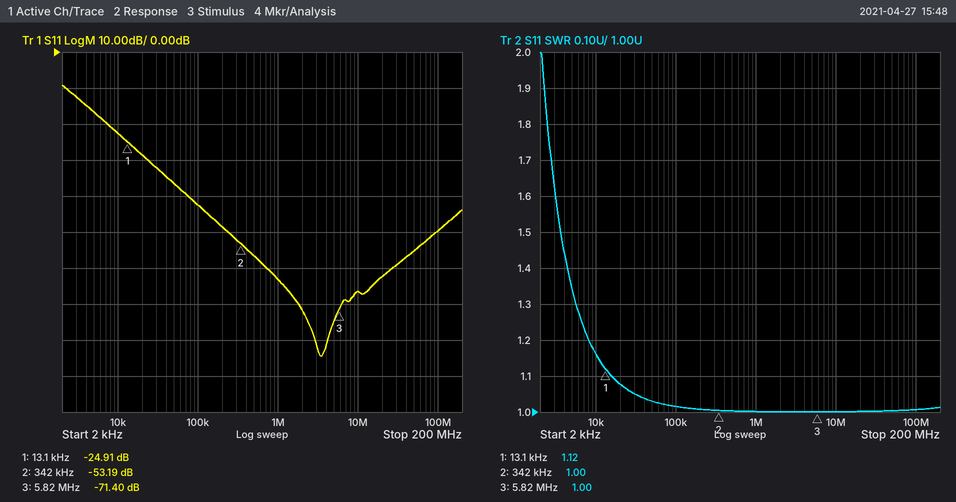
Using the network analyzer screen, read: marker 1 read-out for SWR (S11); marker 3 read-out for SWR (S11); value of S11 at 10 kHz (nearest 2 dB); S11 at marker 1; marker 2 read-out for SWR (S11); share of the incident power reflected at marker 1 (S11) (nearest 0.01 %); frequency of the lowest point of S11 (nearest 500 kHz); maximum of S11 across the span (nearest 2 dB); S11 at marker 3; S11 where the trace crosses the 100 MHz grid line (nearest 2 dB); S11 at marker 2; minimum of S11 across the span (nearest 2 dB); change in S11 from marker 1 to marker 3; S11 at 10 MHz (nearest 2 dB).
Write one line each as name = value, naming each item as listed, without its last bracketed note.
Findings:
marker 1 read-out for SWR = 1.12
marker 3 read-out for SWR = 1.00
value of S11 at 10 kHz = -22 dB
S11 at marker 1 = -24.91 dB
marker 2 read-out for SWR = 1.00
share of the incident power reflected at marker 1 (S11) = 0.32 %
frequency of the lowest point of S11 = 3.5 MHz
maximum of S11 across the span = -10 dB
S11 at marker 3 = -71.40 dB
S11 where the trace crosses the 100 MHz grid line = -50 dB
S11 at marker 2 = -53.19 dB
minimum of S11 across the span = -84 dB
change in S11 from marker 1 to marker 3 = -46.49 dB
S11 at 10 MHz = -66 dB
